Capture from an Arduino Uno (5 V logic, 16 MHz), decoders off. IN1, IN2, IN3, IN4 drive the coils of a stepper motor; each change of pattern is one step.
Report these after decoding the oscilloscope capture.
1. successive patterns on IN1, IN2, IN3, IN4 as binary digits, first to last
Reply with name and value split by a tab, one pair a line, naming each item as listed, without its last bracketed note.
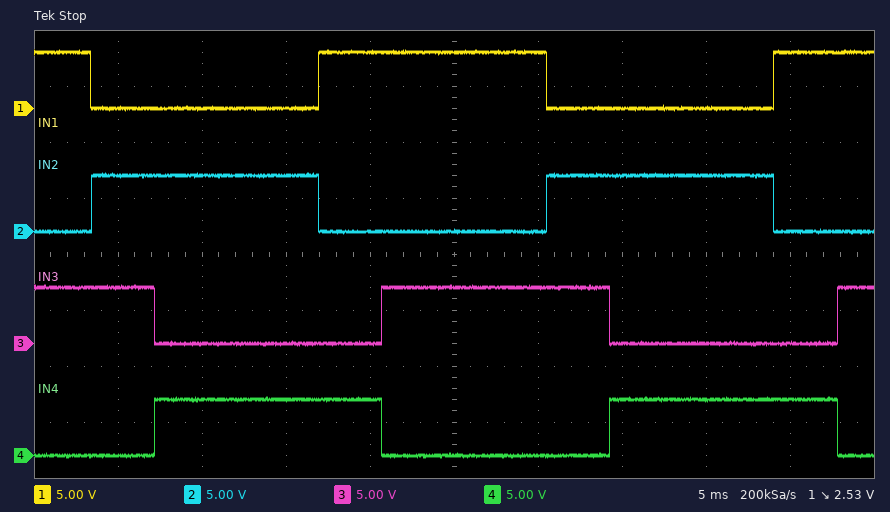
successive patterns on IN1, IN2, IN3, IN4 as binary digits, first to last	1010 0110 0101 1001 1010 0110 0101 1001 1010
